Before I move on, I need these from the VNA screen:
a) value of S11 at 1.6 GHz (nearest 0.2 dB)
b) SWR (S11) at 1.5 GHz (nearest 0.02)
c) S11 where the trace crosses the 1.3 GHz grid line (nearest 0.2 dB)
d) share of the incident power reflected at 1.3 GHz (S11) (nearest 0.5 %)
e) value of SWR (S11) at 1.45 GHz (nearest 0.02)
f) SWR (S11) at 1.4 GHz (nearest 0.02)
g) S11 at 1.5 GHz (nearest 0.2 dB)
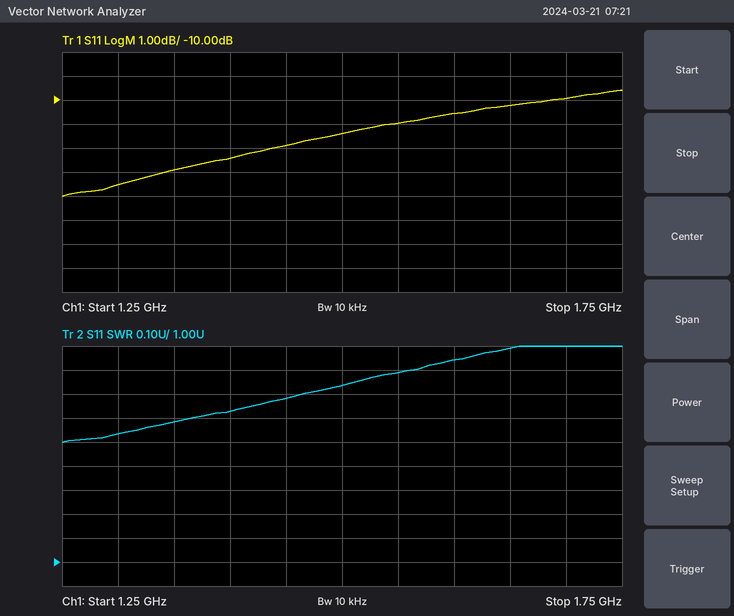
-10.6 dB
1.74
-13.6 dB
4.5 %
1.68
1.62
-11.4 dB
